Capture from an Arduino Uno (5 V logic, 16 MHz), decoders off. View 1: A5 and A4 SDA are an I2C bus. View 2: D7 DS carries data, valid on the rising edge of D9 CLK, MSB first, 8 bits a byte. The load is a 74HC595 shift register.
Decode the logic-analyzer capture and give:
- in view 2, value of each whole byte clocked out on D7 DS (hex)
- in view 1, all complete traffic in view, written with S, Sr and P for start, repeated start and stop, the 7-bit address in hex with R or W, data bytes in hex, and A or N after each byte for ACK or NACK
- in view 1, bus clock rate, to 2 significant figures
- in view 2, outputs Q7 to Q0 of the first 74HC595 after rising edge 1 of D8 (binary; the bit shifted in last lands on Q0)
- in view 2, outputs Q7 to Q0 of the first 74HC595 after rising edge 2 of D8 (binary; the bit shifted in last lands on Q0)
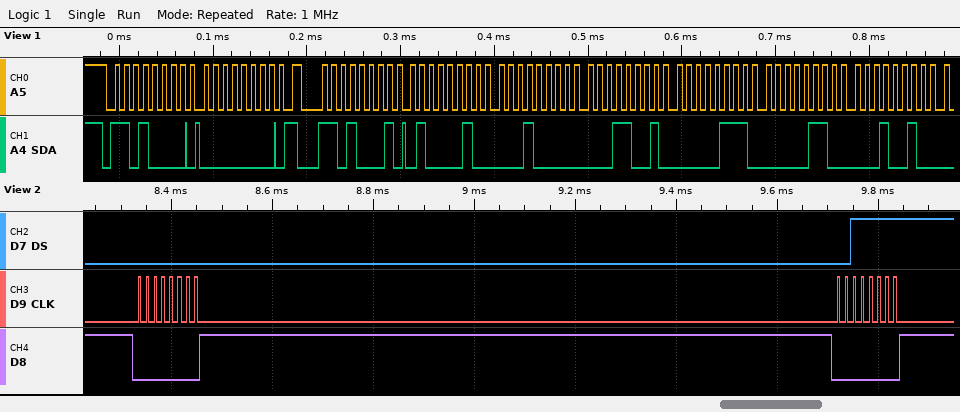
00 3F
S 68W A 00 A Sr 68R A 42 A 10 A 19 A 07 A 06 A 12 A
100 kHz
00000000
00111111
